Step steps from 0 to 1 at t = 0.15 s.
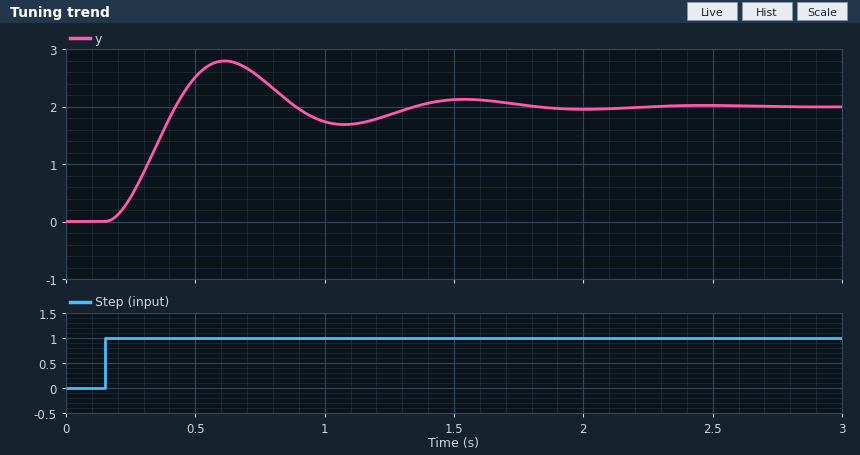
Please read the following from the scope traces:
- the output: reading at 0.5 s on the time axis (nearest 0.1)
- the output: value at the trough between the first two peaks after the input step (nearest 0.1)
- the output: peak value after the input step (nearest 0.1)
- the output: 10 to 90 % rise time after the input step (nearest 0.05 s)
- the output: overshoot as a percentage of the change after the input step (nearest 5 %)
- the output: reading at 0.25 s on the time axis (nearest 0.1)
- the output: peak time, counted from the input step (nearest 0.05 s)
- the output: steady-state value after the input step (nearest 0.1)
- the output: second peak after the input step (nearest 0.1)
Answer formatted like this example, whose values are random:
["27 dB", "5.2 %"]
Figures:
["2.5", "1.7", "2.8", "0.20 s", "40 %", "0.4", "0.45 s", "2.0", "2.1"]
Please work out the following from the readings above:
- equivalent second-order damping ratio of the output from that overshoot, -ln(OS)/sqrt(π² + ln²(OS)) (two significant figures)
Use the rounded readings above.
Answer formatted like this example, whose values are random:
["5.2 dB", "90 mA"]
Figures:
["0.28"]
